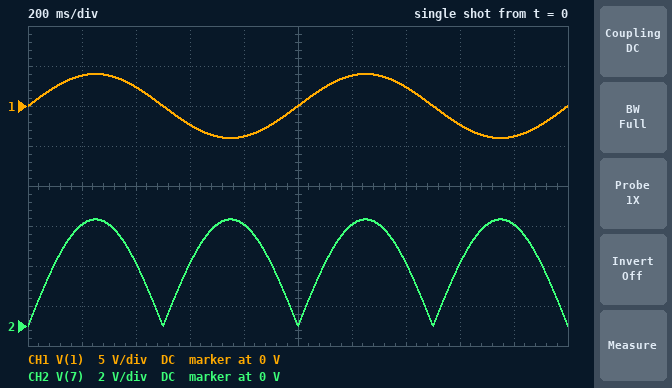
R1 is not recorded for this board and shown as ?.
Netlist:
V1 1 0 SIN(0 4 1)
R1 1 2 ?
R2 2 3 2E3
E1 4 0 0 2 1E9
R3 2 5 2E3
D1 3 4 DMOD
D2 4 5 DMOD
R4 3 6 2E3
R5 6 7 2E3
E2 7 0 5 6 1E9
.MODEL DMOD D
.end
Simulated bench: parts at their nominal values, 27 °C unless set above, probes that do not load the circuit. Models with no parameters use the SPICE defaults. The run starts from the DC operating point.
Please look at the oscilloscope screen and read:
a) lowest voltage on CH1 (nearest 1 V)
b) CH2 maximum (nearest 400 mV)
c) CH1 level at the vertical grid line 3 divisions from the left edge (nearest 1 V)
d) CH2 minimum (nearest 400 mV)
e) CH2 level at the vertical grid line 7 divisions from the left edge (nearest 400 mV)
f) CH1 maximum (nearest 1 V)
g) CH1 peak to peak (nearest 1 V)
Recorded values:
-4 V
5.2 V
-2 V
0 V
3.2 V
4 V
8 V
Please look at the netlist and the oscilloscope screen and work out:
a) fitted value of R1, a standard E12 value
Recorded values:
1.5 kΩ
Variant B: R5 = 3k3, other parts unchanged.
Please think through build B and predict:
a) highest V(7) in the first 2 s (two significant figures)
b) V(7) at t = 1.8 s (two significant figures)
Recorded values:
8.8 V
6.2 V
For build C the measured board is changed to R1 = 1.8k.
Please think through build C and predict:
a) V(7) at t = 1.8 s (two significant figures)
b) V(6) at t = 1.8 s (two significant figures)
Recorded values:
4.2 V
2.8 V
